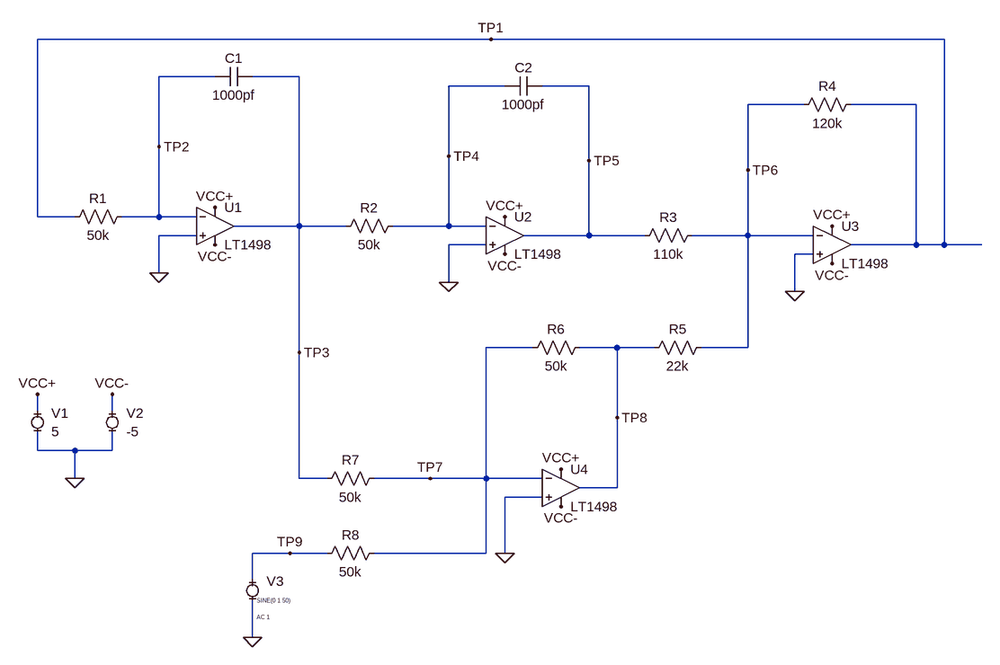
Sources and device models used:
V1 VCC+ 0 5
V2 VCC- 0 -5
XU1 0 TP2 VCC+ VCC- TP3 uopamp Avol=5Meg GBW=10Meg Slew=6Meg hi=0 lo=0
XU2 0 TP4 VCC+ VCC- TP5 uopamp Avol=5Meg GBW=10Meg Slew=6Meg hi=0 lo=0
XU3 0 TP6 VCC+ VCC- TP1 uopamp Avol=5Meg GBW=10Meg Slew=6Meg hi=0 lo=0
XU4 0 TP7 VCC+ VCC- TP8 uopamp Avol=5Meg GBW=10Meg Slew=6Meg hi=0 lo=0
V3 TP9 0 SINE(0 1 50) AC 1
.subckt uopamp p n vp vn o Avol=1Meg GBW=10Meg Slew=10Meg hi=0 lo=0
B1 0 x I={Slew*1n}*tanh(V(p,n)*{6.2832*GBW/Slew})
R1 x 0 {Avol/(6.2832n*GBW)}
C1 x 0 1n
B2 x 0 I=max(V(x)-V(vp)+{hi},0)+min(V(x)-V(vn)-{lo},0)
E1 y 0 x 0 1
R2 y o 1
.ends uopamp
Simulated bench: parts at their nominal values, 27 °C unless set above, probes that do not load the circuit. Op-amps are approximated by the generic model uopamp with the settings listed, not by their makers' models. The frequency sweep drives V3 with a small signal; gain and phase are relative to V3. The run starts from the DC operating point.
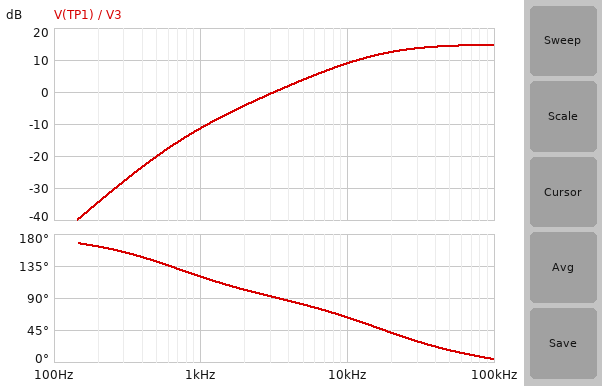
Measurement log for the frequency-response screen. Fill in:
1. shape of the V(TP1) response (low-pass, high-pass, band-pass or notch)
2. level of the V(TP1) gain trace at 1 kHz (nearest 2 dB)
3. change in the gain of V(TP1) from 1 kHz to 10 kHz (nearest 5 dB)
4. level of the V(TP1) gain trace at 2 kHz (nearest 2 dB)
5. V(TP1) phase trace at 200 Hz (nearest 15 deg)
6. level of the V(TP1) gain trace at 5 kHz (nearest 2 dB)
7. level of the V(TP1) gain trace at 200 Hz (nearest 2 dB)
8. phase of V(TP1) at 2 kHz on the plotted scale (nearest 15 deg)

high-pass
-12 dB
20 dB
-4 dB
165 deg
4 dB
-34 dB
105 deg
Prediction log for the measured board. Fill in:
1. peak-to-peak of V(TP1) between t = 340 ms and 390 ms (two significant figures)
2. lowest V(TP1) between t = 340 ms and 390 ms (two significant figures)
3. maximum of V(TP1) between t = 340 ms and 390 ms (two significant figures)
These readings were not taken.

2.5 mV
-1.2 mV
1.2 mV
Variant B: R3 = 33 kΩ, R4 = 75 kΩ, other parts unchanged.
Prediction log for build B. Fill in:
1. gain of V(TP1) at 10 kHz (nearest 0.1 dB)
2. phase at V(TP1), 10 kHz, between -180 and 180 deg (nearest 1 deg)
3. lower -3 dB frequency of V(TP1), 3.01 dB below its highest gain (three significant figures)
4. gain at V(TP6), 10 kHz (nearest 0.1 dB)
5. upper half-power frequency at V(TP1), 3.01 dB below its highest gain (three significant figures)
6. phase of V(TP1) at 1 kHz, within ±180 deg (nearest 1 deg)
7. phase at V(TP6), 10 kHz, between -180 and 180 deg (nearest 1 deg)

8.2 dB
54 deg
8.85 kHz
-51.8 dB
1.29 MHz
154 deg
-36 deg
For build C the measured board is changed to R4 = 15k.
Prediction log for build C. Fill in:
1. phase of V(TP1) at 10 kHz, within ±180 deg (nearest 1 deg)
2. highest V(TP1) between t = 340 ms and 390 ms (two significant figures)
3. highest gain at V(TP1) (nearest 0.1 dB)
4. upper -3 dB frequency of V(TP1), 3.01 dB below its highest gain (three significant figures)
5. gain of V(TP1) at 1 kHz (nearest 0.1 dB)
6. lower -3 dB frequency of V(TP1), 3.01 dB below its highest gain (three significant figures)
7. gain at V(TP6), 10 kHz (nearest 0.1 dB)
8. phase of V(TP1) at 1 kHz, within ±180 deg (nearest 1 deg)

12 deg
1.2 mV
-3.3 dB
2.64 MHz
-10.2 dB
1.63 kHz
-63.4 dB
100 deg
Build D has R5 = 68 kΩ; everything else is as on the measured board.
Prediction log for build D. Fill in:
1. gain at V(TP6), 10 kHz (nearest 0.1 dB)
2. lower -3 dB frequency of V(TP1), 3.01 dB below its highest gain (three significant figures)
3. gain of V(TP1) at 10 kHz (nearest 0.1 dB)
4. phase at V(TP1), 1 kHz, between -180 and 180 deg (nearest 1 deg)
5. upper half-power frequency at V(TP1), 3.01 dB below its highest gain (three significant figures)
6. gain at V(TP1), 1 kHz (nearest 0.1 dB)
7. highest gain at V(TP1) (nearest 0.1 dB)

-55.5 dB
4.10 kHz
4.5 dB
151 deg
1.87 MHz
-16.3 dB
5.0 dB
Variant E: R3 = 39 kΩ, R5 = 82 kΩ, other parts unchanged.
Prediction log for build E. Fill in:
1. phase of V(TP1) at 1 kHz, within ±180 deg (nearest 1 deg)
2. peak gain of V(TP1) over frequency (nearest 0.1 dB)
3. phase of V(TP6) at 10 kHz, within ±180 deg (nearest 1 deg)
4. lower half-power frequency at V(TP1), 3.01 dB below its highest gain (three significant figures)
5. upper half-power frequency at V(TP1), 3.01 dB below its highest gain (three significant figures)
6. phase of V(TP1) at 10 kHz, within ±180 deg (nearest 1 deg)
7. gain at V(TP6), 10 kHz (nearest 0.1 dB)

171 deg
5.8 dB
-56 deg
4.71 kHz
594 kHz
34 deg
-55.0 dB
